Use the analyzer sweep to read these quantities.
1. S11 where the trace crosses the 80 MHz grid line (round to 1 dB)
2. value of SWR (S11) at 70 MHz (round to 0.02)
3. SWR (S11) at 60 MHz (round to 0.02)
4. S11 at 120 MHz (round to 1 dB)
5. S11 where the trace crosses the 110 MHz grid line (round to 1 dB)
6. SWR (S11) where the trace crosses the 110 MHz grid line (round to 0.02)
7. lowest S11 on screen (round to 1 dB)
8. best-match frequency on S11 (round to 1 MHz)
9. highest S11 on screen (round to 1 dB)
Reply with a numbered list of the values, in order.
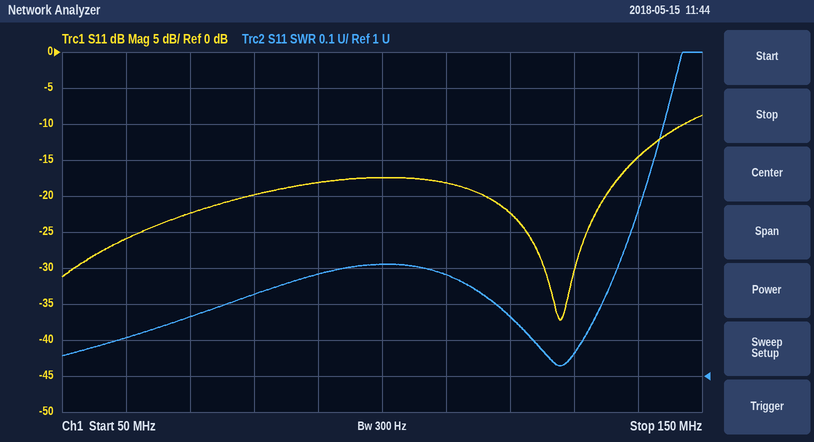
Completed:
1. -20 dB
2. 1.16
3. 1.10
4. -22 dB
5. -18 dB
6. 1.28
7. -37 dB
8. 128 MHz
9. -9 dB
